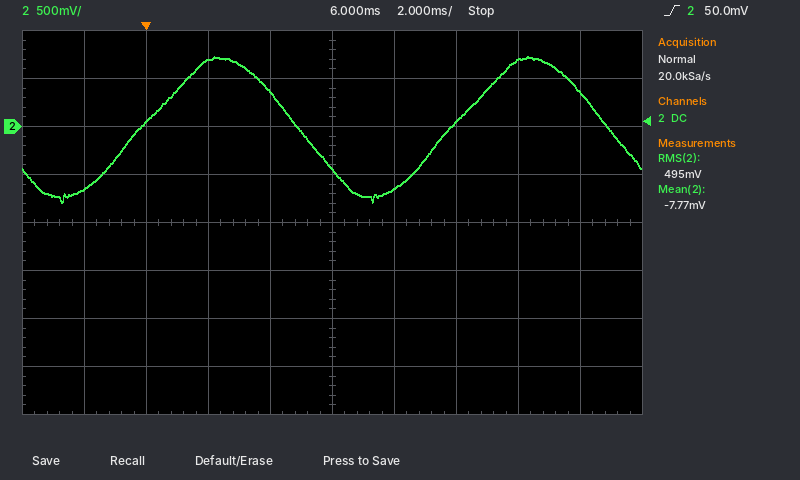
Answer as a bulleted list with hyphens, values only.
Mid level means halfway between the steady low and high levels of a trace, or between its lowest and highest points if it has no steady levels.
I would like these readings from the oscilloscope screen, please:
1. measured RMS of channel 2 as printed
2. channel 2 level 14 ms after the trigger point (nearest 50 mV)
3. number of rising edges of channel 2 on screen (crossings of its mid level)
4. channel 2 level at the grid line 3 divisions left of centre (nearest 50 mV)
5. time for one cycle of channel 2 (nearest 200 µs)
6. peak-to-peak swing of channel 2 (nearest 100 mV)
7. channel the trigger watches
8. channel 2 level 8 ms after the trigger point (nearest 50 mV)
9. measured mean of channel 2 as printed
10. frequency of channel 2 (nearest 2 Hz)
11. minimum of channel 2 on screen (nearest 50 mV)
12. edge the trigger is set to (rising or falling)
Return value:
- 495 mV
- 350 mV
- 2
- 50 mV
- 10.0 ms
- 1.50 V
- channel 2
- -650 mV
- -7.77 mV
- 100 Hz
- -800 mV
- rising
